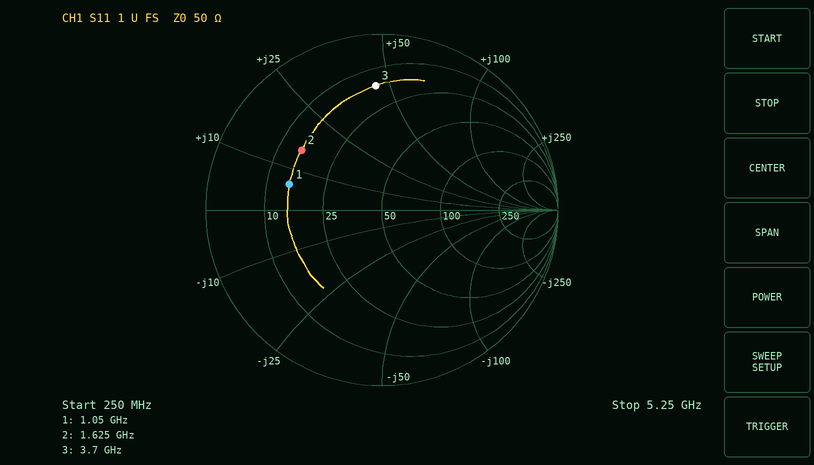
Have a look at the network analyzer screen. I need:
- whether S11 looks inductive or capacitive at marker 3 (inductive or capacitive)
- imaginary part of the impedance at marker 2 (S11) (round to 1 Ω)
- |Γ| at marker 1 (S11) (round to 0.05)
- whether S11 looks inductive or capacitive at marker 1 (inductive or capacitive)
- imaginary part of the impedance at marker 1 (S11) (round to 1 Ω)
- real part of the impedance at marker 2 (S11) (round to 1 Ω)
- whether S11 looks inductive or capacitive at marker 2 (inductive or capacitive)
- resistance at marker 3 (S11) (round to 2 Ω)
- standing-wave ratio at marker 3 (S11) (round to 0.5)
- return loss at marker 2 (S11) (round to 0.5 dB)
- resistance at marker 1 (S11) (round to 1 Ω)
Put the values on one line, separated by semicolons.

inductive; +15 Ω; 0.55; inductive; +6 Ω; 15 Ω; inductive; 16 Ω; 6.0; 5.0 dB; 15 Ω
